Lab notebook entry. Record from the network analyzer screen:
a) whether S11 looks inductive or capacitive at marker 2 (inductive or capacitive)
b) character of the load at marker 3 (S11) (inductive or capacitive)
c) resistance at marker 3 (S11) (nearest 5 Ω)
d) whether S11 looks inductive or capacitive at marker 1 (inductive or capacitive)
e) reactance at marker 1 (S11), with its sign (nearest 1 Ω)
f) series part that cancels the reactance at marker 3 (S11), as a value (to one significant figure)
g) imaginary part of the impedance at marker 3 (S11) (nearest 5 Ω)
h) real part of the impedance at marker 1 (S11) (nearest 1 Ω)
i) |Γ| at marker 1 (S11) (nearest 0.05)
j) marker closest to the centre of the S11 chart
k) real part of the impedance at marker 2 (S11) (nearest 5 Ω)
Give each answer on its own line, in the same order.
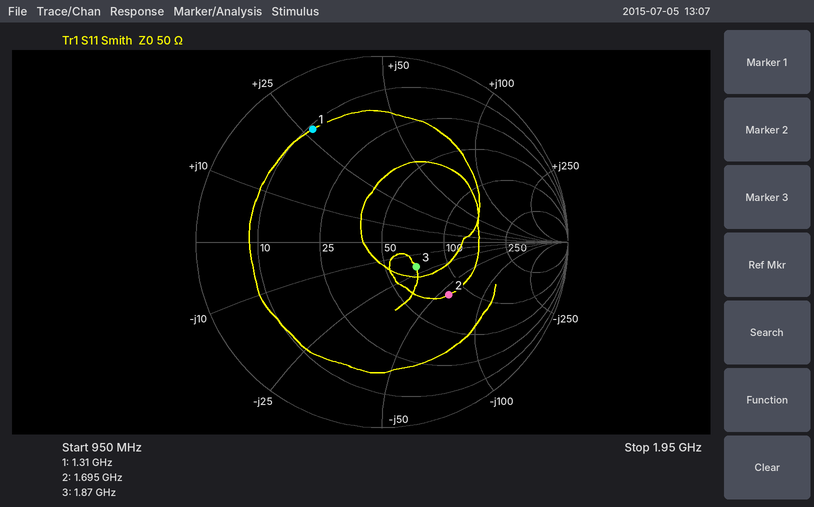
capacitive
capacitive
70 Ω
inductive
+27 Ω
2 nH
-20 Ω
11 Ω
0.70
marker 3
80 Ω
